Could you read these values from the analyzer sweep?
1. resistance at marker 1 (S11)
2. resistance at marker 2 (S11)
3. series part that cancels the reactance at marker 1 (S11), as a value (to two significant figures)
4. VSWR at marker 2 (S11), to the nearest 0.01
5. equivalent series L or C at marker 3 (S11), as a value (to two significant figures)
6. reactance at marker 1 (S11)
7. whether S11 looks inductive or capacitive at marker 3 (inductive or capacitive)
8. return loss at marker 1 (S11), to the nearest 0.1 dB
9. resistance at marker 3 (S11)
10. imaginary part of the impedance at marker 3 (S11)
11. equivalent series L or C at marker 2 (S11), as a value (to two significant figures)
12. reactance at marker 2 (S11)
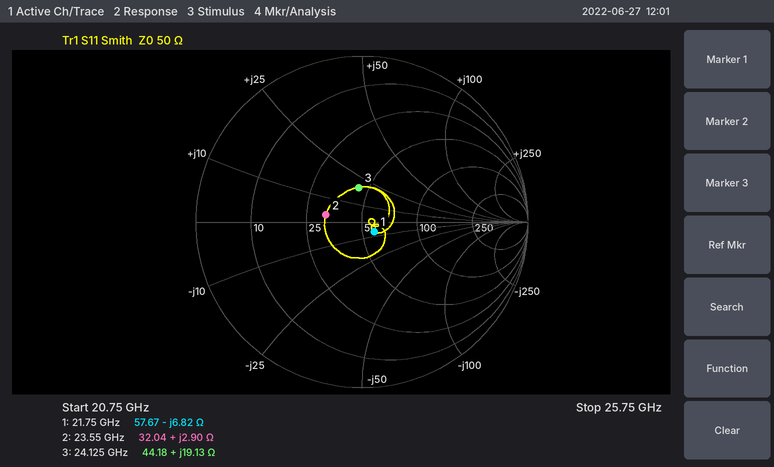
57.67 Ω
32.04 Ω
50 pH
1.57
130 pH
-6.82 Ω
inductive
20.4 dB
44.18 Ω
+19.13 Ω
20 pH
+2.90 Ω
